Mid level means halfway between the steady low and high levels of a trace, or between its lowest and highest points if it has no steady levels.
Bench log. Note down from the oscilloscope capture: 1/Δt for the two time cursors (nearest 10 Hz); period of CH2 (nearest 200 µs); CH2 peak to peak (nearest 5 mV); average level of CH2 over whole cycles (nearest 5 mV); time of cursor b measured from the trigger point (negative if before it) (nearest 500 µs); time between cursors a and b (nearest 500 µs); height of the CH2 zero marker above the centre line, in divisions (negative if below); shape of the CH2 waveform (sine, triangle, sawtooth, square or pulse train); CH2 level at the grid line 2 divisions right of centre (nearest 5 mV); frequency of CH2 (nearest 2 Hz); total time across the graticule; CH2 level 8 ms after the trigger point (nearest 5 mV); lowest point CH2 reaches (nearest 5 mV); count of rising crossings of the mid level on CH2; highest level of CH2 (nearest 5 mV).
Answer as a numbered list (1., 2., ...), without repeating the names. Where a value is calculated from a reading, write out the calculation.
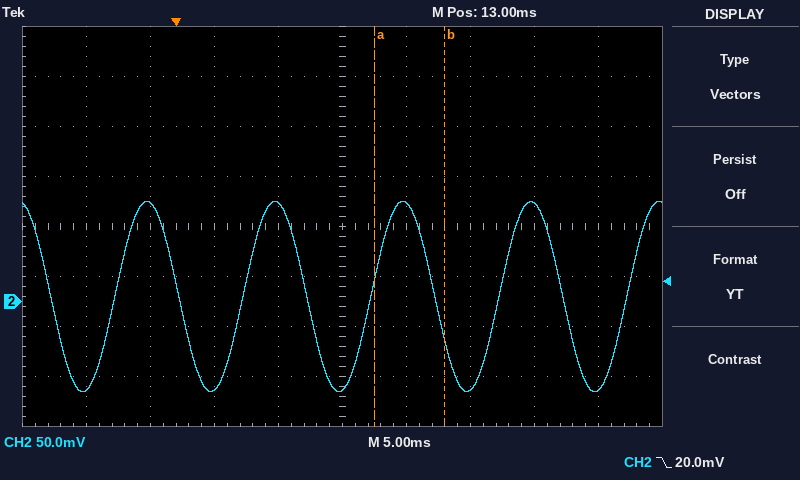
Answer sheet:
1. 1 / 5.5 ms ≈ 180 Hz
2. 10.0 ms
3. 100 mV − (-90 mV) = 190 mV
4. (100 mV + (-90 mV)) / 2 ≈ 5 mV
5. +21.0 ms
6. 5.5 ms
7. -1.5 div
8. sine
9. -90 mV
10. 1 / 10.0 ms ≈ 100 Hz
11. 50 ms
12. 100 mV
13. -90 mV
14. 5
15. 100 mV
